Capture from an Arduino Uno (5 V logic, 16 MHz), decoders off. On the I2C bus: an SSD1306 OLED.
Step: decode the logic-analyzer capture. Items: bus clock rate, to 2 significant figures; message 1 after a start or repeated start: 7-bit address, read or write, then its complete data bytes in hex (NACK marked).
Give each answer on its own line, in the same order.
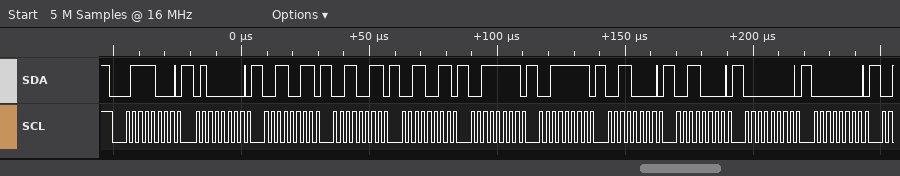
400 kHz
0x3C write: 40 33 33 33 3F 3F 30 30 00 00
